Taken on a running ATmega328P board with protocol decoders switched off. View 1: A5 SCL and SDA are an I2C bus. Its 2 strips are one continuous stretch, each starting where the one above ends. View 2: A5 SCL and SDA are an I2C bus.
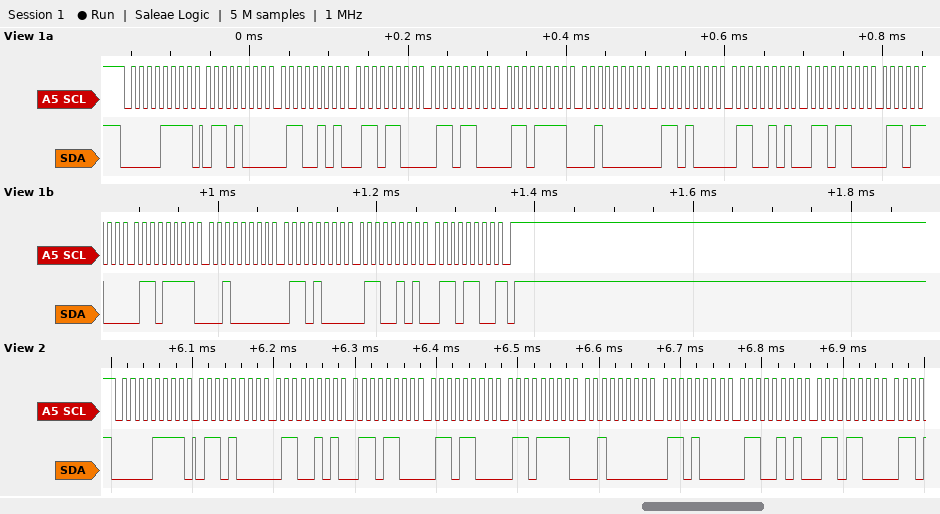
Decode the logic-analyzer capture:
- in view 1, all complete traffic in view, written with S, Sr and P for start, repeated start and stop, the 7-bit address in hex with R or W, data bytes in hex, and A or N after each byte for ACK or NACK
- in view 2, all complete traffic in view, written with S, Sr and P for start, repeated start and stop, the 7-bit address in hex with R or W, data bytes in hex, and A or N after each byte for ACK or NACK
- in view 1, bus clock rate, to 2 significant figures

S 07R A 68 A 65 A 6C A 6C A 6F A 20 A 68 A 65 A 6C A 6C A 6F A 20 A 68 A 65 A 6C N P
S 07R A 68 A 65 A 6C A 6C A 6F A 20 A 68 A 65 A 6C A
100 kHz
